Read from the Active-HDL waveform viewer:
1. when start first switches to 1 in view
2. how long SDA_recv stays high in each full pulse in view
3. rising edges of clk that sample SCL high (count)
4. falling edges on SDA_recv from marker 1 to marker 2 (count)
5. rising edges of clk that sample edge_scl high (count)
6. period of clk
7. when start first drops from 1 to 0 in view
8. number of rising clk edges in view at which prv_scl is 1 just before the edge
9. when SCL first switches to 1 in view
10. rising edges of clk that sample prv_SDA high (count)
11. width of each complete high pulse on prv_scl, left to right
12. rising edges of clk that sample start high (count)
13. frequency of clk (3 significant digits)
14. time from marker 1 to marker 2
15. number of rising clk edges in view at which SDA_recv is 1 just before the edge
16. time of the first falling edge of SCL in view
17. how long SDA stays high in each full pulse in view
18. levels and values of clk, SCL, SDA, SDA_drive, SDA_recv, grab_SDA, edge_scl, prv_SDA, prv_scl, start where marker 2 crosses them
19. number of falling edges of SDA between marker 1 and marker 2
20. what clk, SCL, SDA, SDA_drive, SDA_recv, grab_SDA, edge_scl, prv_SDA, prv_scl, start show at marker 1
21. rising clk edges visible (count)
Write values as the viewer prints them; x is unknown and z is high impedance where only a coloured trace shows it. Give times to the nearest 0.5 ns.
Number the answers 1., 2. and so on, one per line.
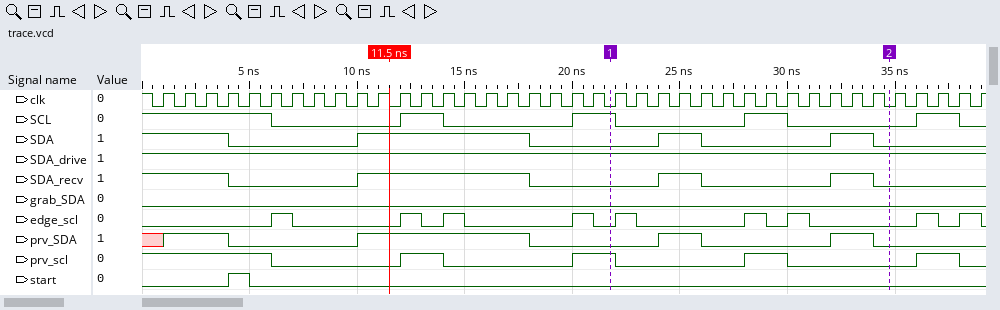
1. 4 ns
2. 8 ns, 2 ns, 2 ns
3. 14
4. 2
5. 9
6. 1 ns
7. 5 ns
8. 14
9. 12 ns
10. 15
11. 2 ns, 2 ns, 2 ns, 2 ns
12. 1
13. 1.00 GHz
14. 13 ns
15. 16
16. 6 ns
17. 8 ns, 2 ns, 2 ns
18. clk=0, SCL=0, SDA=0, SDA_drive=1, SDA_recv=0, grab_SDA=0, edge_scl=0, prv_SDA=0, prv_scl=0, start=0
19. 2
20. clk=0, SCL=1, SDA=0, SDA_drive=1, SDA_recv=0, grab_SDA=0, edge_scl=0, prv_SDA=0, prv_scl=1, start=0
21. 39
